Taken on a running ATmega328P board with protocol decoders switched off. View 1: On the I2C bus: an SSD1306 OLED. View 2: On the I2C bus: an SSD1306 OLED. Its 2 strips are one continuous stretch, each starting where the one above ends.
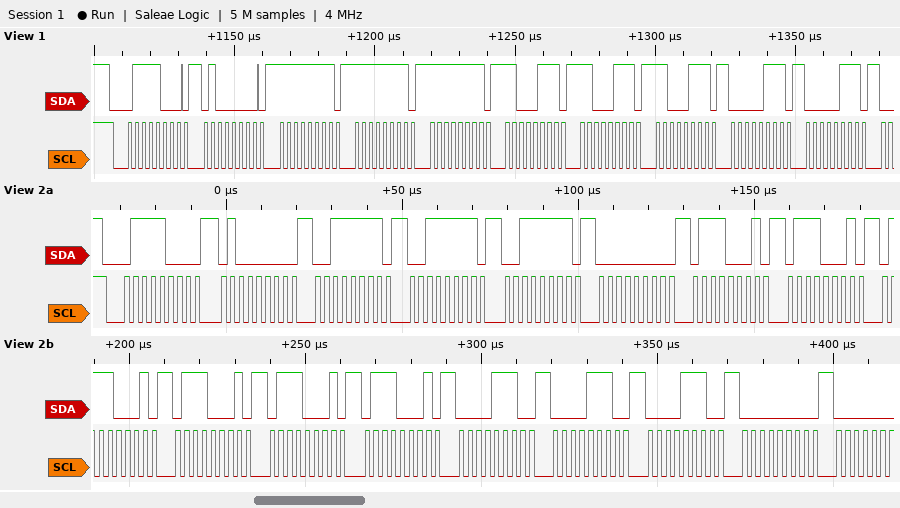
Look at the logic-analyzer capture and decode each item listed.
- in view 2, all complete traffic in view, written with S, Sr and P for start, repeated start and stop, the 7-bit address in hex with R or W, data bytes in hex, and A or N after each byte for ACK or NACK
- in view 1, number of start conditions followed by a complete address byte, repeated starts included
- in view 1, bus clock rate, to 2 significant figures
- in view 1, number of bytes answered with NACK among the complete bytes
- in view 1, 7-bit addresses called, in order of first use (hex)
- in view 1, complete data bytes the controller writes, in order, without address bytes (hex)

S 3CW A 40 A 3F A 3F A 3F A 00 A 71 A 71 A 71 A 71 A 71 A 71 A 0E A 0E A 0E A 00 A
1
400 kHz
0
0x3C
40 FF FF FF C7 C7 C7 07 07
